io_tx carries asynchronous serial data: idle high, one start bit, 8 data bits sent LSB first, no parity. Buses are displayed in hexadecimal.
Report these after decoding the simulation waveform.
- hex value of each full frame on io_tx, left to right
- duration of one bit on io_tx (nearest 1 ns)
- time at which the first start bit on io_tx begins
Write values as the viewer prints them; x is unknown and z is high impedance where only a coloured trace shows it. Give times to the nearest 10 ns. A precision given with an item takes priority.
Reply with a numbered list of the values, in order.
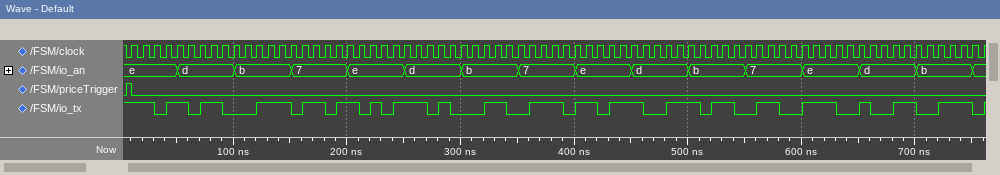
1. 1B, 5B, 31, 3B, 33, 32
2. 10 ns
3. 30 ns
